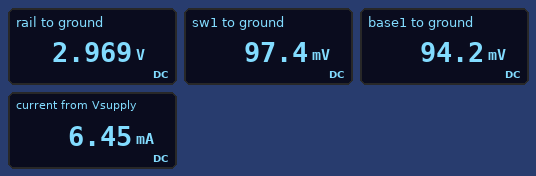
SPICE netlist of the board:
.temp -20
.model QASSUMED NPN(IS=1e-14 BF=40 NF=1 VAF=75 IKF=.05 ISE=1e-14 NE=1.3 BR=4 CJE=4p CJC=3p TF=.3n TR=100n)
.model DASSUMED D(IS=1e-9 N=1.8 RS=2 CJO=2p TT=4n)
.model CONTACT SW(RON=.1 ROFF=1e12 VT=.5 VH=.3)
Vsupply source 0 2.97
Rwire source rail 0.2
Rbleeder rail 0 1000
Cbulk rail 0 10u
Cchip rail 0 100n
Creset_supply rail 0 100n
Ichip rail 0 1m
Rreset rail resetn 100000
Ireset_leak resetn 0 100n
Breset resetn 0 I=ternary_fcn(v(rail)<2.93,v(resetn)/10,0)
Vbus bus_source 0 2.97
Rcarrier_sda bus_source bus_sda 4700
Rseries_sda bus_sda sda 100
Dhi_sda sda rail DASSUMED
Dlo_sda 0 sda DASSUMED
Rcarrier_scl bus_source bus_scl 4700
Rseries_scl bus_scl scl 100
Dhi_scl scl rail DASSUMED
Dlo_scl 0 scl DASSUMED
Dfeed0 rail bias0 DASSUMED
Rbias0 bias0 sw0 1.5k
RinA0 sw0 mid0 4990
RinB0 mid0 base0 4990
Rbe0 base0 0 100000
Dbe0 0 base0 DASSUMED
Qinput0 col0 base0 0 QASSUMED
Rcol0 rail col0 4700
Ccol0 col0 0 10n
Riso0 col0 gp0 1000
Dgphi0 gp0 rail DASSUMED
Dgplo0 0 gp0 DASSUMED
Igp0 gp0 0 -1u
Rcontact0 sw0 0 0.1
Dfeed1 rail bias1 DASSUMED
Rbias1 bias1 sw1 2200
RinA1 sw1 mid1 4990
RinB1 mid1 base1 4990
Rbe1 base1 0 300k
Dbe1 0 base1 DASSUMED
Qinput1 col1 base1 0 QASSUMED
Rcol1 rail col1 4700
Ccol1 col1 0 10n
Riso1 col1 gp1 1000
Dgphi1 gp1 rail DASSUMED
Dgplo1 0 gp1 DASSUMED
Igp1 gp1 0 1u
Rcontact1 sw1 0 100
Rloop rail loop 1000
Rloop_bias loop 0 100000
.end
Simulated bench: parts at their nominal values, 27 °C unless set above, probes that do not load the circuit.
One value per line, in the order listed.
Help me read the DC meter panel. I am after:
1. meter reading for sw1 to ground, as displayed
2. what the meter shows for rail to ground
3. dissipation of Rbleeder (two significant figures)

97.4 mV
2.969 V
8.8 mW
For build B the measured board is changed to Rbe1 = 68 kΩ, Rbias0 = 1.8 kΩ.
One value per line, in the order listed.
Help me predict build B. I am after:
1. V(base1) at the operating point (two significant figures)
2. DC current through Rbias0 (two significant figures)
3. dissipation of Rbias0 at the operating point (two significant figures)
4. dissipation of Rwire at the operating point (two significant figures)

85 mV
1.2 mA
2.8 mW
7.7 µW
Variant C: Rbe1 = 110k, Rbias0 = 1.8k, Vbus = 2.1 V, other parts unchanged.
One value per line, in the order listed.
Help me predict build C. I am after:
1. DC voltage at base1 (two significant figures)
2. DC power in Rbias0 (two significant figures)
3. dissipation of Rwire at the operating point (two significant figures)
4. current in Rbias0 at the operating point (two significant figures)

89 mV
2.8 mW
7.7 µW
1.2 mA
